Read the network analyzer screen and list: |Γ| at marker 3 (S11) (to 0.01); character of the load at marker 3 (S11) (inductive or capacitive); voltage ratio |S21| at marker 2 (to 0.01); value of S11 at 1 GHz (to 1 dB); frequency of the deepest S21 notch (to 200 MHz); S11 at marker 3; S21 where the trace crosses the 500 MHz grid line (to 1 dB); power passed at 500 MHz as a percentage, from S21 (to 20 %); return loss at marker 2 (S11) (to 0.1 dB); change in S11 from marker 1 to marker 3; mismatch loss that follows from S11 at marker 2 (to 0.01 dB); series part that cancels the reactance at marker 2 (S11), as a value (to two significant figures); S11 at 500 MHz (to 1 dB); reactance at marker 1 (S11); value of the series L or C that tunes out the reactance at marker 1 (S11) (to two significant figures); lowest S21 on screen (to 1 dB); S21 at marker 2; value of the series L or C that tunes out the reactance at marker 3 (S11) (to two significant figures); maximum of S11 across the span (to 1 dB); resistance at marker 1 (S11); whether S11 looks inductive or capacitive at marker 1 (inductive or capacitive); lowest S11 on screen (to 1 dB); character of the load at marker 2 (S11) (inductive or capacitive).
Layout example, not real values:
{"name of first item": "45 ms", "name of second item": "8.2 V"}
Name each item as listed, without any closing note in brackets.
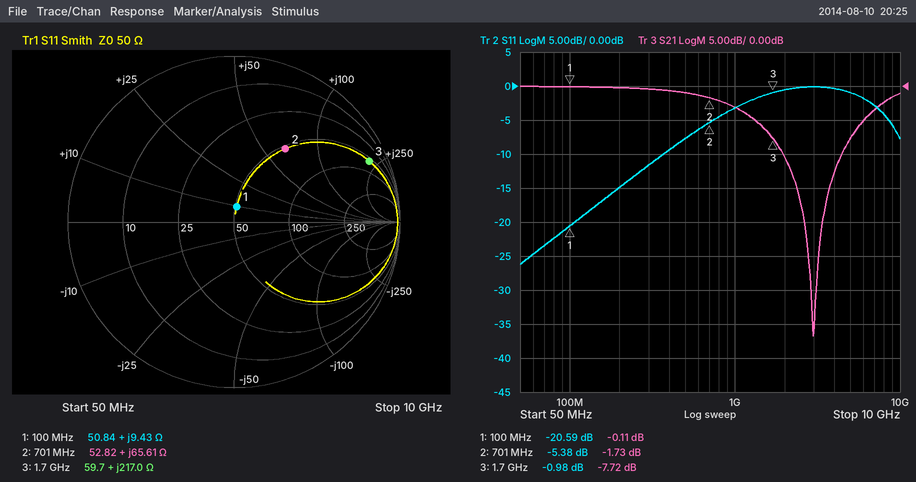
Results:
{"|Γ| at marker 3 (S11)": "0.89", "character of the load at marker 3 (S11)": "inductive", "voltage ratio |S21| at marker 2": "0.82", "value of S11 at 1 GHz": "-3 dB", "frequency of the deepest S21 notch": "3.0 GHz", "S11 at marker 3": "-0.98 dB", "S21 where the trace crosses the 500 MHz grid line": "-1 dB", "power passed at 500 MHz as a percentage, from S21": "80 %", "return loss at marker 2 (S11)": "5.4 dB", "change in S11 from marker 1 to marker 3": "19.61 dB", "mismatch loss that follows from S11 at marker 2": "1.49 dB", "series part that cancels the reactance at marker 2 (S11), as a value": "3.5 pF", "S11 at 500 MHz": "-8 dB", "reactance at marker 1": "+9.43 Ω", "value of the series L or C that tunes out the reactance at marker 1 (S11)": "170 pF", "lowest S21 on screen": "-37 dB", "S21 at marker 2": "-1.73 dB", "value of the series L or C that tunes out the reactance at marker 3 (S11)": "430 fF", "maximum of S11 across the span": "0 dB", "resistance at marker 1": "50.84 Ω", "whether S11 looks inductive or capacitive at marker 1": "inductive", "lowest S11 on screen": "-26 dB", "character of the load at marker 2 (S11)": "inductive"}
